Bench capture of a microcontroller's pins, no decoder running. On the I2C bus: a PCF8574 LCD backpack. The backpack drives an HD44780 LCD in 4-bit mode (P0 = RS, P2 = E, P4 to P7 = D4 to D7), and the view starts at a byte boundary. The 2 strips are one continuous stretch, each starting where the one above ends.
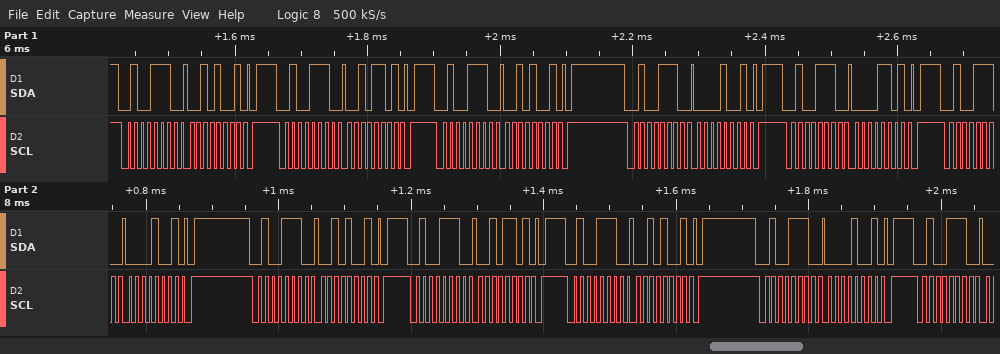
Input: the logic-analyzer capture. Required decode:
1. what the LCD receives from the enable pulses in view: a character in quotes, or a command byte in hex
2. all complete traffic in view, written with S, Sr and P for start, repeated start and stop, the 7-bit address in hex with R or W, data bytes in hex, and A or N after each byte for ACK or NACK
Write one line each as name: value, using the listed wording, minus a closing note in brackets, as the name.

what the LCD receives from the enable pulses in view: a character in quotes, or a command byte in hex: ' '
all complete traffic in view, written with S, Sr and P for start, repeated start and stop, the 7-bit address in hex with R or W, data bytes in hex, and A or N after each byte for ACK or NACK: S 27W A 29 A P S 27W A 2D A P S 27W A 29 A P S 27W A 09 A P S 27W A 0D A P S 27W A 09 A P S 27W A 29 A P S 27W A 2D A P S 27W A 29 A P S 27W A 09 A P S 27W A
